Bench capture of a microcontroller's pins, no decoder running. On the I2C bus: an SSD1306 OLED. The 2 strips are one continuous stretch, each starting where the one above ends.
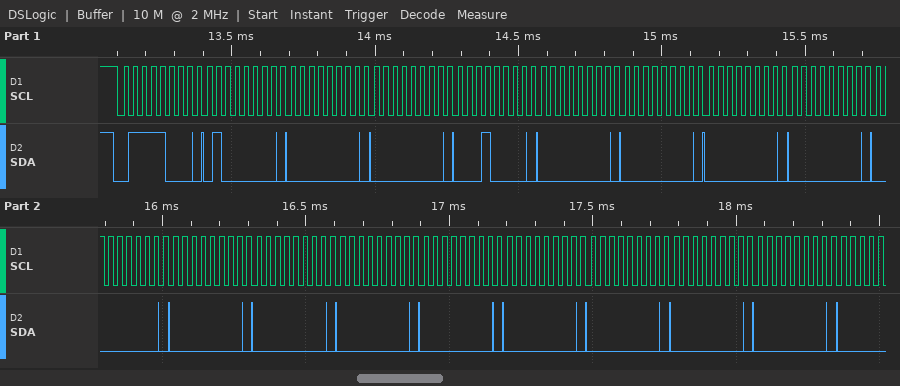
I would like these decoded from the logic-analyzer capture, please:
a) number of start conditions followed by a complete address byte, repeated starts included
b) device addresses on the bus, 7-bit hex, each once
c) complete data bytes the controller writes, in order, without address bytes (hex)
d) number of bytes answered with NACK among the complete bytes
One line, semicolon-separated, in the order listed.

1; 0x3C; 40 00 00 10 00 00 00 00 00 00 00 00 00 00 00 00 00; 0
